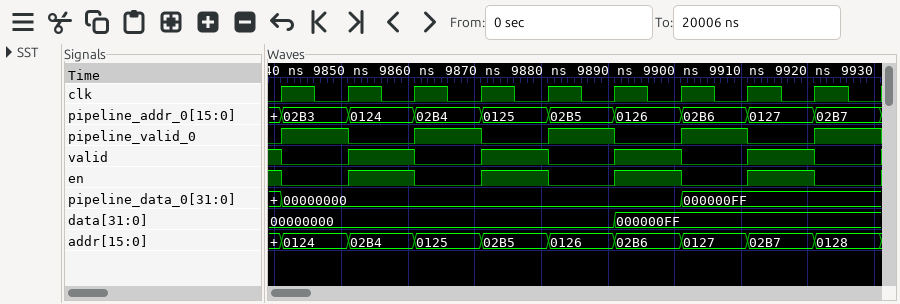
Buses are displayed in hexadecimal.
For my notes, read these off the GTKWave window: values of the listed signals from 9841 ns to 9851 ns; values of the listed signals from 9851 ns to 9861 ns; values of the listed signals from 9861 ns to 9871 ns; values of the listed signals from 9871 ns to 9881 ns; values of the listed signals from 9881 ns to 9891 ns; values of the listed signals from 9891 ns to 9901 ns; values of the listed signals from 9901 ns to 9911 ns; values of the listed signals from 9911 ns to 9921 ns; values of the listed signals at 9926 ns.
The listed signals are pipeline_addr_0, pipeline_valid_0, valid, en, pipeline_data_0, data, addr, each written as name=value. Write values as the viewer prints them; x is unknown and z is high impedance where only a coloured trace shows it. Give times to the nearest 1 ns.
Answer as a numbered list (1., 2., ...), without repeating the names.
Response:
1. pipeline_addr_0=02B3, pipeline_valid_0=1, valid=0, en=0, pipeline_data_0=00000000, data=00000000, addr=0124
2. pipeline_addr_0=0124, pipeline_valid_0=0, valid=1, en=1, pipeline_data_0=00000000, data=00000000, addr=02B4
3. pipeline_addr_0=02B4, pipeline_valid_0=1, valid=0, en=0, pipeline_data_0=00000000, data=00000000, addr=0125
4. pipeline_addr_0=0125, pipeline_valid_0=0, valid=1, en=1, pipeline_data_0=00000000, data=00000000, addr=02B5
5. pipeline_addr_0=02B5, pipeline_valid_0=1, valid=0, en=0, pipeline_data_0=00000000, data=00000000, addr=0126
6. pipeline_addr_0=0126, pipeline_valid_0=0, valid=1, en=1, pipeline_data_0=00000000, data=000000FF, addr=02B6
7. pipeline_addr_0=02B6, pipeline_valid_0=1, valid=0, en=0, pipeline_data_0=000000FF, data=000000FF, addr=0127
8. pipeline_addr_0=0127, pipeline_valid_0=0, valid=1, en=1, pipeline_data_0=000000FF, data=000000FF, addr=02B7
9. pipeline_addr_0=02B7, pipeline_valid_0=1, valid=0, en=0, pipeline_data_0=000000FF, data=000000FF, addr=0128
